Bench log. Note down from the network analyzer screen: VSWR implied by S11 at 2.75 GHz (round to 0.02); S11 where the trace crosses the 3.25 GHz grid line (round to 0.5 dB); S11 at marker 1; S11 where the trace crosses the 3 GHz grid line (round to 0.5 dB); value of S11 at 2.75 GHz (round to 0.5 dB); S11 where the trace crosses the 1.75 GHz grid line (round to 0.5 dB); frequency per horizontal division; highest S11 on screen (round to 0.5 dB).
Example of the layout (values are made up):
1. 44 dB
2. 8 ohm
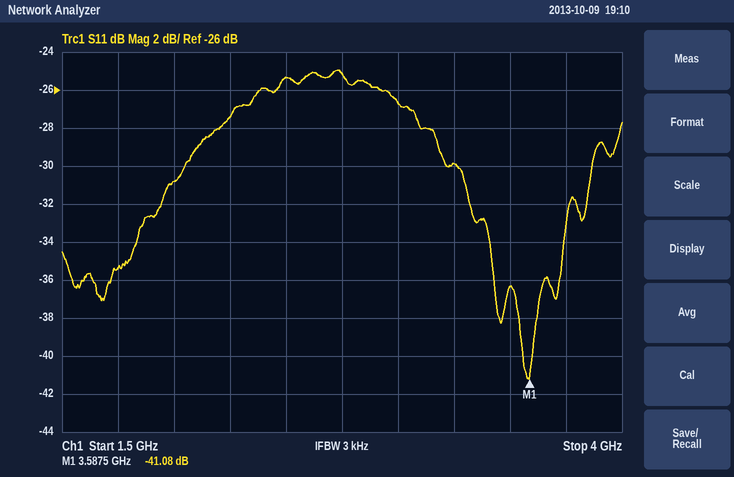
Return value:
1. 1.12
2. -30.0 dB
3. -41.08 dB
4. -26.5 dB
5. -25.0 dB
6. -35.5 dB
7. 250 MHz
8. -25.0 dB
